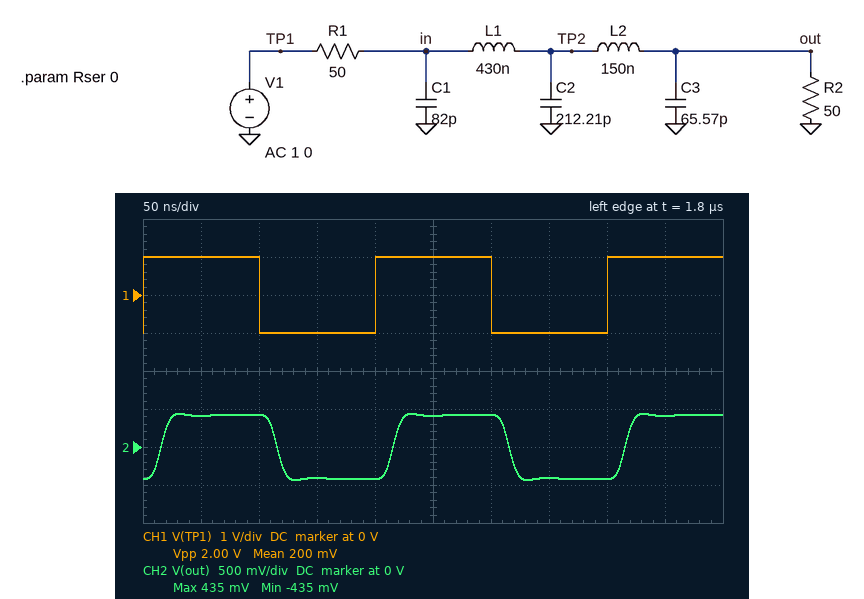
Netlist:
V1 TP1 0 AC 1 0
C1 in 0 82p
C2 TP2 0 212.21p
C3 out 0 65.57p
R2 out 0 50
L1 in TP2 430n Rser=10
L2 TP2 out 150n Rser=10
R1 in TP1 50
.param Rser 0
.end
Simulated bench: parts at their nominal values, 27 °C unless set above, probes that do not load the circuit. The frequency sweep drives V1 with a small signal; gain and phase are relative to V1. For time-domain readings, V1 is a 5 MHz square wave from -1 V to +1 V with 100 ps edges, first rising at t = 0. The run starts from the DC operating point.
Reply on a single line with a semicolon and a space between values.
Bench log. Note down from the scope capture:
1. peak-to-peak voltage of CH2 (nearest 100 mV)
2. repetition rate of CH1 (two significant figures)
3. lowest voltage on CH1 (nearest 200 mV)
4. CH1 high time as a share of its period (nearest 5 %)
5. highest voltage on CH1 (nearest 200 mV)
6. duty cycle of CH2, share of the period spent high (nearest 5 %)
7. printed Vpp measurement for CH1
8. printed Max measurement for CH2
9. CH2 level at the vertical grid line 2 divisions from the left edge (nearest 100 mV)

900 mV; 5.0 MHz; -1.0 V; 50 %; 1.0 V; 50 %; 2.00 V; 435 mV; 400 mV
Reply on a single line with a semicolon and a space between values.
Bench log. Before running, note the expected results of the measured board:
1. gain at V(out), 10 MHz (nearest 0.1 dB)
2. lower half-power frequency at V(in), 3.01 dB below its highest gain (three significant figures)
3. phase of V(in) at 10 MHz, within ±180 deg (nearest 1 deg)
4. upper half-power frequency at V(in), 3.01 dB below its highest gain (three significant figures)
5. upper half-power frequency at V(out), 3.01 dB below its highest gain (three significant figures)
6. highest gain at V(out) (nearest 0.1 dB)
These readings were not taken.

-8.0 dB; 22.2 MHz; -8 deg; 64.3 MHz; 26.9 MHz; -7.6 dB
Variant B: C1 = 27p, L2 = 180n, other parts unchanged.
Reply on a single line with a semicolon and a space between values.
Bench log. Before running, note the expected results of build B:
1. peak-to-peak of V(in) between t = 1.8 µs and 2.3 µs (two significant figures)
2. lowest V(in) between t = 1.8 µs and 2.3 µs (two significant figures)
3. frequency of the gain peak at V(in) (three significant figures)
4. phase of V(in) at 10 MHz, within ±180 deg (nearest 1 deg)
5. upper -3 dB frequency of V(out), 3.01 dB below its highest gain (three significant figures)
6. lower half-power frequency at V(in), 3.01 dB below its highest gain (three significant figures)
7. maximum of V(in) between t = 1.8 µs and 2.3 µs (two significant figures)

2.0 V; -1.0 V; 57.5 MHz; -3 deg; 25.4 MHz; 27.5 MHz; 1.0 V
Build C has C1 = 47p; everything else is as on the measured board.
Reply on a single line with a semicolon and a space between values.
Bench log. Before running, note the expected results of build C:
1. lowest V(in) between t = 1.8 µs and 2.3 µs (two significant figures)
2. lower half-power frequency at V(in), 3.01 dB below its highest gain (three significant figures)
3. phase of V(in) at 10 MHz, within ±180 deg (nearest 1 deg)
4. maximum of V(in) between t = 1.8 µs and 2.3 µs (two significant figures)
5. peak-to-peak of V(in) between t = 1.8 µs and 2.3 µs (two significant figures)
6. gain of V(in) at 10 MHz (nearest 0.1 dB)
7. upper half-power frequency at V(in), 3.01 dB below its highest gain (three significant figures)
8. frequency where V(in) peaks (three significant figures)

-880 mV; 24.9 MHz; -5 deg; 880 mV; 1.8 V; -6.4 dB; 93.6 MHz; 45.2 MHz
